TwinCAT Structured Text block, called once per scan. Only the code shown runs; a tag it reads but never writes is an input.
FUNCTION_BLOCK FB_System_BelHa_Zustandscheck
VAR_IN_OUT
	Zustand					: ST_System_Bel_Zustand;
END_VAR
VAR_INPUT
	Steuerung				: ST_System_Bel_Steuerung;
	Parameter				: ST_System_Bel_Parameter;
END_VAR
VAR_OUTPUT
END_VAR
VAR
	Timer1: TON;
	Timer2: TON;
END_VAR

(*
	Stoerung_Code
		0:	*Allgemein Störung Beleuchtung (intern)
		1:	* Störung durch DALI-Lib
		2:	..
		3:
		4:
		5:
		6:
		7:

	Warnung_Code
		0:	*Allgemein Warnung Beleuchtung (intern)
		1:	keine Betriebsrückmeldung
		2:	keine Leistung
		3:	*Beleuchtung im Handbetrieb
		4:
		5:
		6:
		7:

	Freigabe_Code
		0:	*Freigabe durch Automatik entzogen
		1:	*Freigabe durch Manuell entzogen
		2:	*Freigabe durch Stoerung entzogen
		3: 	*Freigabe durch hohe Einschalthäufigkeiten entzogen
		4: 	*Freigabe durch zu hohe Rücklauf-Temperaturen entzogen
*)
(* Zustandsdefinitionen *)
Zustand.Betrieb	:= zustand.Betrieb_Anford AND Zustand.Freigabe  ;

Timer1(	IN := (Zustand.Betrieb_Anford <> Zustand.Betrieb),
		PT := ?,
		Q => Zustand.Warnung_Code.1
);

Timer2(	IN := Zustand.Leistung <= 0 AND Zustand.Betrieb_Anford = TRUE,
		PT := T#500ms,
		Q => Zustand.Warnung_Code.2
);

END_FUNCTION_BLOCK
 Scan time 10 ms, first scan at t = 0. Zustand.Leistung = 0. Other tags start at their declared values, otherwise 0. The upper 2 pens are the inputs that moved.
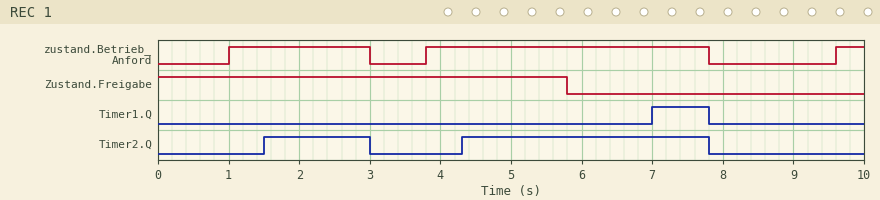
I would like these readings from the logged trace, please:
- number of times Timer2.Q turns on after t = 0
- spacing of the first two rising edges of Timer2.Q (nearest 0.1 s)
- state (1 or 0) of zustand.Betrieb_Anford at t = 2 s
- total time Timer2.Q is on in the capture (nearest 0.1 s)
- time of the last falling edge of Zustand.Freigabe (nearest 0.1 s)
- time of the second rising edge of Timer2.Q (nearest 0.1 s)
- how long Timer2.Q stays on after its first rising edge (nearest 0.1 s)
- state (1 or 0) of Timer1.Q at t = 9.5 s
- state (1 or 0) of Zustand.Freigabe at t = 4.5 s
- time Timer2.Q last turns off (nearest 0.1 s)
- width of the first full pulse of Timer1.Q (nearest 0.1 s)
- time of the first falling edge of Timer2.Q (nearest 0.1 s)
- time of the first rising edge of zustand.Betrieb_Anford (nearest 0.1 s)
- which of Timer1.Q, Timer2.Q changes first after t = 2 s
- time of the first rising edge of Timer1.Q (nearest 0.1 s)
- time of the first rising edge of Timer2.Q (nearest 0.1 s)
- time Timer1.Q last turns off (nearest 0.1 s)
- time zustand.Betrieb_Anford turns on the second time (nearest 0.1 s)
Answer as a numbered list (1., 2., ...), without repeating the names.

1. 2
2. 2.8 s
3. 1
4. 5.0 s
5. 5.8 s
6. 4.3 s
7. 1.5 s
8. 0
9. 1
10. 7.8 s
11. 0.8 s
12. 3.0 s
13. 1.0 s
14. Timer2.Q
15. 7.0 s
16. 1.5 s
17. 7.8 s
18. 3.8 s
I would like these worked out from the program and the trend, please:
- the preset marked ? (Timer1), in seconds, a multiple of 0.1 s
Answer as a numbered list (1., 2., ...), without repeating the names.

1. 1.2 s
